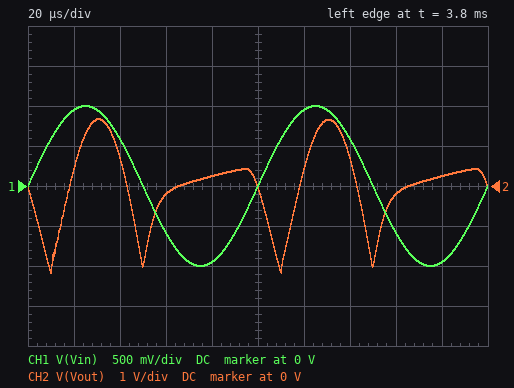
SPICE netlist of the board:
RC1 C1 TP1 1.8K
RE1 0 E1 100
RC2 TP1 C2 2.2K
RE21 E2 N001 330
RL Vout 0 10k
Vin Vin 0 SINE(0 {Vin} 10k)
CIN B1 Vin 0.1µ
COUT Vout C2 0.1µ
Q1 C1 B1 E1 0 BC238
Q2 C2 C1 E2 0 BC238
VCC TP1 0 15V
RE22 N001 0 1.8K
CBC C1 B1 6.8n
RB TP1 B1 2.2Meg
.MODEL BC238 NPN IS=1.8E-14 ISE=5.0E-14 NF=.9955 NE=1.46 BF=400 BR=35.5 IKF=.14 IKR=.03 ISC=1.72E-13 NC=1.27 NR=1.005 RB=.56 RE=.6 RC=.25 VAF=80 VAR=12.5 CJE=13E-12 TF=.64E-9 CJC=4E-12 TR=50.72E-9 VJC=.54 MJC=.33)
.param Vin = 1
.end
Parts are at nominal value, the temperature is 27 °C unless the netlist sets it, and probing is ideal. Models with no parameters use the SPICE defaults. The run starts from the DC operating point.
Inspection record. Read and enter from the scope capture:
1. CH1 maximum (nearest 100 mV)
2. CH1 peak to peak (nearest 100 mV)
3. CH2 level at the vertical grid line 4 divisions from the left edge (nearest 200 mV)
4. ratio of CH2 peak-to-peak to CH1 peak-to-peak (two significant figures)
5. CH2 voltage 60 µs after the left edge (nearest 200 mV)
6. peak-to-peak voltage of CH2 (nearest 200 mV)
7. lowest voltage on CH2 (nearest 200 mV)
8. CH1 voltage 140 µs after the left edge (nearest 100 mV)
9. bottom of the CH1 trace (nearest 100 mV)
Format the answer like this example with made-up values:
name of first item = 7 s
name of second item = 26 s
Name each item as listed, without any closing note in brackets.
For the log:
CH1 maximum = 1.0 V
CH1 peak to peak = 2.0 V
CH2 level at the vertical grid line 4 divisions from the left edge = 200 mV
ratio of CH2 peak-to-peak to CH1 peak-to-peak = 1.9
CH2 voltage 60 µs after the left edge = -200 mV
peak-to-peak voltage of CH2 = 3.8 V
lowest voltage on CH2 = -2.2 V
CH1 voltage 140 µs after the left edge = 600 mV
bottom of the CH1 trace = -1.0 V
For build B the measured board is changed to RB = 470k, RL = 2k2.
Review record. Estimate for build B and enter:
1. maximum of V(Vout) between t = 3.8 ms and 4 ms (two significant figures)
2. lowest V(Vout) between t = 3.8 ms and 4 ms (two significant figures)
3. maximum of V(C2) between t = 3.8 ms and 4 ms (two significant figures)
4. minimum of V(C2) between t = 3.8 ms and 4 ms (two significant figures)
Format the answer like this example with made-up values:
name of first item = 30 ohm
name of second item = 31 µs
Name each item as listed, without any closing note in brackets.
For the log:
maximum of V(Vout) between t = 3.8 ms and 4 ms = 2.1 V
lowest V(Vout) between t = 3.8 ms and 4 ms = -2.1 V
maximum of V(C2) between t = 3.8 ms and 4 ms = 13 V
minimum of V(C2) between t = 3.8 ms and 4 ms = 8.3 V
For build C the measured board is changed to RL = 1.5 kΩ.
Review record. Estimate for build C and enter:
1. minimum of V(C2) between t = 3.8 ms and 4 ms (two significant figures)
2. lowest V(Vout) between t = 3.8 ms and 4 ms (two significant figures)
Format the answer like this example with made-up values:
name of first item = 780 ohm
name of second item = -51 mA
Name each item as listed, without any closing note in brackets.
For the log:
minimum of V(C2) between t = 3.8 ms and 4 ms = 8.3 V
lowest V(Vout) between t = 3.8 ms and 4 ms = -1.4 V
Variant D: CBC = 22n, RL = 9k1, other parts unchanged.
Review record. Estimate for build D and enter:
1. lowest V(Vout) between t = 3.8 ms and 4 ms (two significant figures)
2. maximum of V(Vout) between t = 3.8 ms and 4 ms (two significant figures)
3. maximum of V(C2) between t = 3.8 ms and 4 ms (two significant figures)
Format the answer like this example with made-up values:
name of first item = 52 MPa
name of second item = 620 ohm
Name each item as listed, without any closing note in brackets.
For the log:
lowest V(Vout) between t = 3.8 ms and 4 ms = -1.2 V
maximum of V(Vout) between t = 3.8 ms and 4 ms = 1.3 V
maximum of V(C2) between t = 3.8 ms and 4 ms = 10 V
